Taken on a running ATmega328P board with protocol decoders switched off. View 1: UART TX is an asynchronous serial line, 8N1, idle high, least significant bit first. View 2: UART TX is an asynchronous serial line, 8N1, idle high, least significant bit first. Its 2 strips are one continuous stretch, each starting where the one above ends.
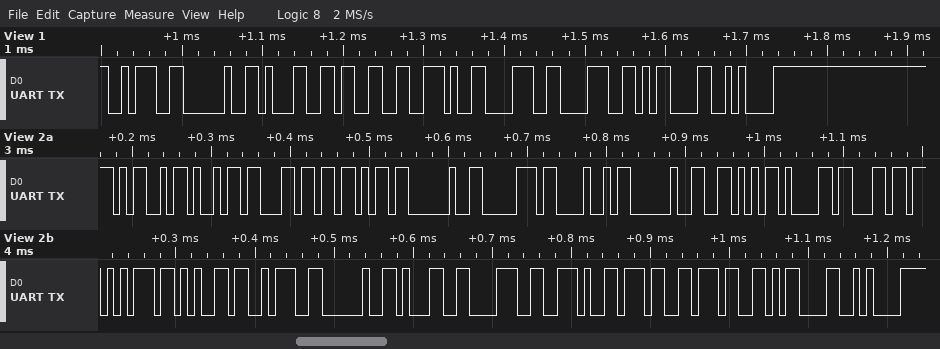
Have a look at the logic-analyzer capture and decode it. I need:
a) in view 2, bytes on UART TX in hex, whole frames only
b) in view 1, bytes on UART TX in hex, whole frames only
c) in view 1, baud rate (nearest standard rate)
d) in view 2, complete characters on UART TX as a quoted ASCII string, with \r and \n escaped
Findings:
0x4D 0x69 0x6C 0x6B 0x20 0x70 0x48 0x20 0x56 0x61 0x6C 0x75 0x65 0x3A 0x20 0x31 0x38 0x2E 0x37 0x37 0x0D 0x0A
3A 20 31 33 2E 38 38 0D 0A
115200 baud
"Milk pH Value: 18.77\r\n"
